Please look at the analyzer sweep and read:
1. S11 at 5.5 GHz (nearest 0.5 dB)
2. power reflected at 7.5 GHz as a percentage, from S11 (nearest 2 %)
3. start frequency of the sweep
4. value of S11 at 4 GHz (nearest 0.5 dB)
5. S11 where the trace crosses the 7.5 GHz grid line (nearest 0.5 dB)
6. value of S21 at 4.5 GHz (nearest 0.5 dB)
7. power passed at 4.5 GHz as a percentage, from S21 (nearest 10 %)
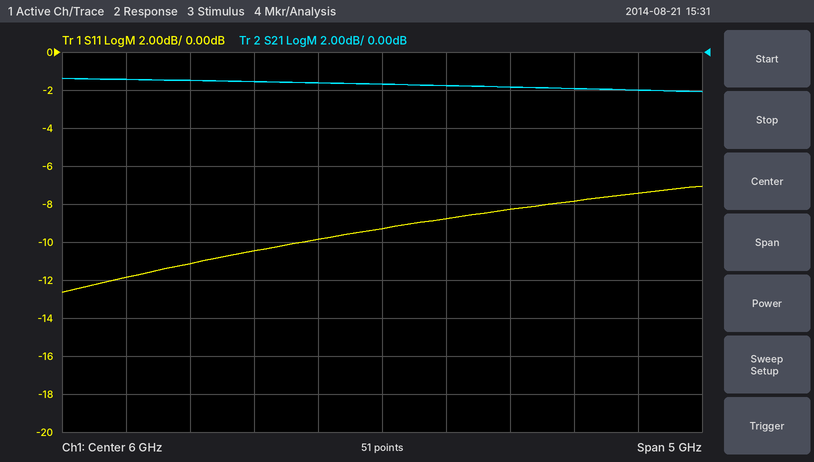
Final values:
-10.0 dB
16 %
3.5 GHz
-12.0 dB
-8.0 dB
-1.5 dB
70 %
